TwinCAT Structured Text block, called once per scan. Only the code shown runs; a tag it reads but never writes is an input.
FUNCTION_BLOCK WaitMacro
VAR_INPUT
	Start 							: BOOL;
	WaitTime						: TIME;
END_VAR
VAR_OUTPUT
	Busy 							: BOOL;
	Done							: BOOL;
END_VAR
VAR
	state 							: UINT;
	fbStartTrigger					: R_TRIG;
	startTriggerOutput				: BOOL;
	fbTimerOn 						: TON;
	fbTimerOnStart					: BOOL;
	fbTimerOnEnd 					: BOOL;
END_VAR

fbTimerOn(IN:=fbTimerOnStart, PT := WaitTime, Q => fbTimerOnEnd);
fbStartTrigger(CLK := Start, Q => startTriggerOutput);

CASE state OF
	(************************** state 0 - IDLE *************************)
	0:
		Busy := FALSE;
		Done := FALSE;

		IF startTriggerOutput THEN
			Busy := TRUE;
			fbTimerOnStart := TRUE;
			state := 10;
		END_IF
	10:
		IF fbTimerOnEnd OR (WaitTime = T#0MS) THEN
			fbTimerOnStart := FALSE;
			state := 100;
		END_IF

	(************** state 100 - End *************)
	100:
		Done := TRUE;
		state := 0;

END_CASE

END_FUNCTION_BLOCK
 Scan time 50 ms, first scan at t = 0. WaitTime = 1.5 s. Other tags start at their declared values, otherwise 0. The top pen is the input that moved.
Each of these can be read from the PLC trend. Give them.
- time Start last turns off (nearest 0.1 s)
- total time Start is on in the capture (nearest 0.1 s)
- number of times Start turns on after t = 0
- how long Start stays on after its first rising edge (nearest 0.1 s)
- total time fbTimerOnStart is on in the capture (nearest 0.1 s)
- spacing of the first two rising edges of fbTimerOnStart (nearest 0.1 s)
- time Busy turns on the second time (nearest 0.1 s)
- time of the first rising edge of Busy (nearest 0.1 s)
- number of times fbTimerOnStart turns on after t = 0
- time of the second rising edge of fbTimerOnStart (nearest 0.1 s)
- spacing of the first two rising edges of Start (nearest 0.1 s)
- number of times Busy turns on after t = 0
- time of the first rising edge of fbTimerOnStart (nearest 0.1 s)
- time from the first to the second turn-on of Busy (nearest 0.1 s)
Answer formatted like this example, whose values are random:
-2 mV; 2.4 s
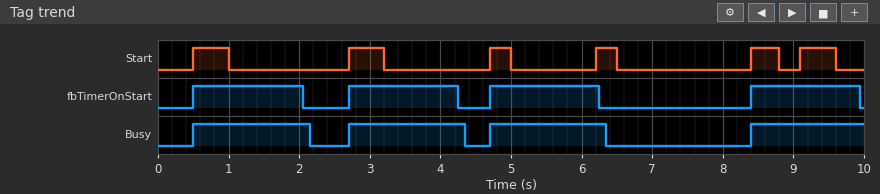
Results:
9.6 s; 2.5 s; 6; 0.5 s; 6.2 s; 2.2 s; 2.7 s; 0.5 s; 4; 2.7 s; 2.2 s; 4; 0.5 s; 2.2 s
